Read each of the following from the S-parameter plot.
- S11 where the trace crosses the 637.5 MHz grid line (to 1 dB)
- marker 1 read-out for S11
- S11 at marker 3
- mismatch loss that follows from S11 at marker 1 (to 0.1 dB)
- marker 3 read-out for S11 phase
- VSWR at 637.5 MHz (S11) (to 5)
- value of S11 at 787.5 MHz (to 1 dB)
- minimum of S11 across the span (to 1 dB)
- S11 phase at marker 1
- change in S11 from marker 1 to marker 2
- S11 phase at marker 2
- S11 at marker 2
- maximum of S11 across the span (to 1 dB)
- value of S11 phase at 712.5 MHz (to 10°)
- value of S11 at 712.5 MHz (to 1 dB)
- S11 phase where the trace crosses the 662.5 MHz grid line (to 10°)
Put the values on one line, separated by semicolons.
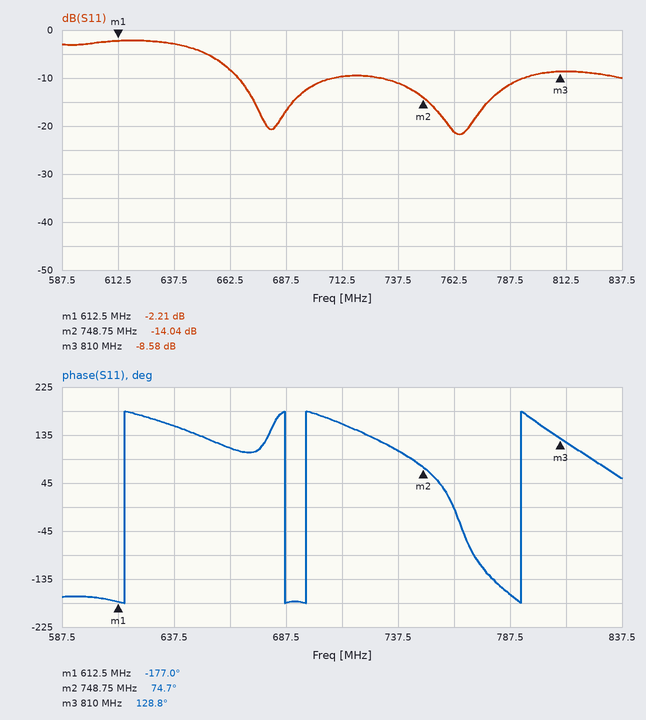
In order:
-3 dB; -2.21 dB; -8.58 dB; 4.0 dB; 128.8°; 5; -11 dB; -22 dB; -177.0°; -11.83 dB; 74.7°; -14.04 dB; -2 dB; 160°; -10 dB; 110°
